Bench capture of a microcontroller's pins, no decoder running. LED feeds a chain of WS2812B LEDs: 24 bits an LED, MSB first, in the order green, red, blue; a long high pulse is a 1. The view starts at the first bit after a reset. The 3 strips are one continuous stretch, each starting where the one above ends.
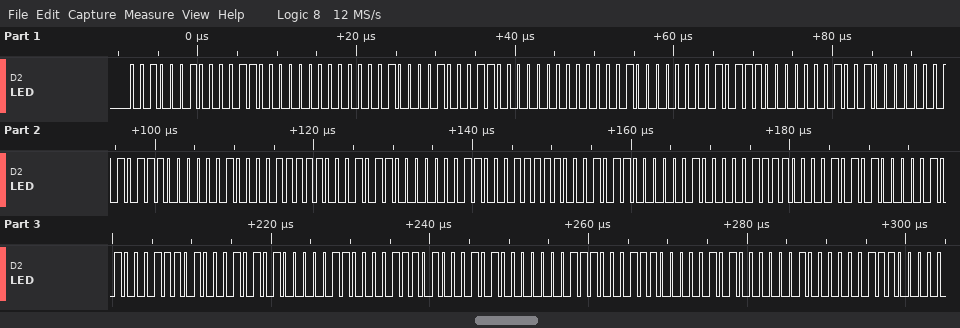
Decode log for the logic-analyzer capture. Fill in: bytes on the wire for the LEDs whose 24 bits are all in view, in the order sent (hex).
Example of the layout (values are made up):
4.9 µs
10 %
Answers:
22 18 00 21 18 00 20 17 01 20 17 02 1F 16 03 1F 16 04 1E 15 05 1D 15 06 1D 14 07 1C 14 08
